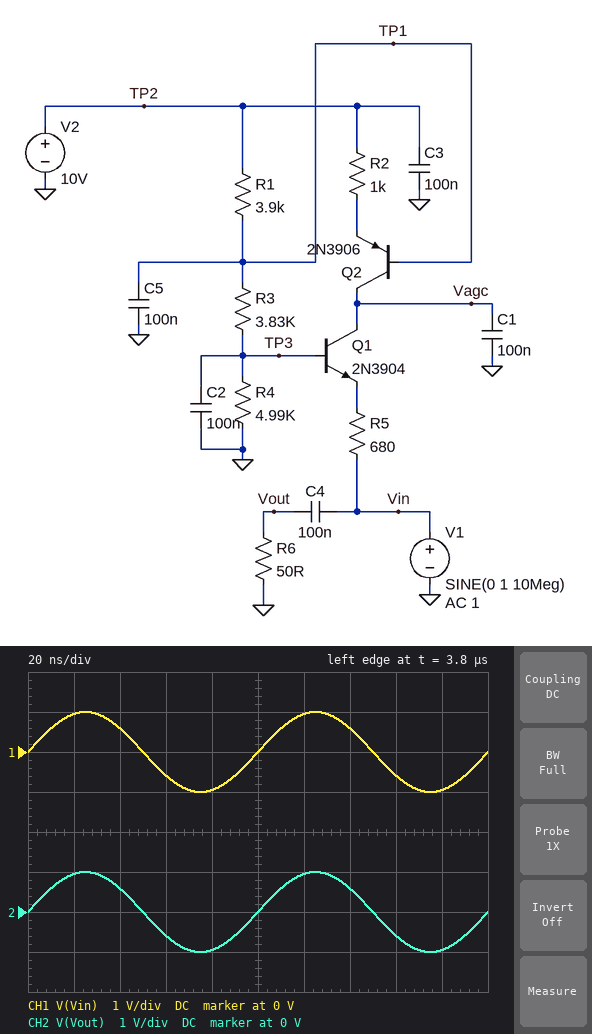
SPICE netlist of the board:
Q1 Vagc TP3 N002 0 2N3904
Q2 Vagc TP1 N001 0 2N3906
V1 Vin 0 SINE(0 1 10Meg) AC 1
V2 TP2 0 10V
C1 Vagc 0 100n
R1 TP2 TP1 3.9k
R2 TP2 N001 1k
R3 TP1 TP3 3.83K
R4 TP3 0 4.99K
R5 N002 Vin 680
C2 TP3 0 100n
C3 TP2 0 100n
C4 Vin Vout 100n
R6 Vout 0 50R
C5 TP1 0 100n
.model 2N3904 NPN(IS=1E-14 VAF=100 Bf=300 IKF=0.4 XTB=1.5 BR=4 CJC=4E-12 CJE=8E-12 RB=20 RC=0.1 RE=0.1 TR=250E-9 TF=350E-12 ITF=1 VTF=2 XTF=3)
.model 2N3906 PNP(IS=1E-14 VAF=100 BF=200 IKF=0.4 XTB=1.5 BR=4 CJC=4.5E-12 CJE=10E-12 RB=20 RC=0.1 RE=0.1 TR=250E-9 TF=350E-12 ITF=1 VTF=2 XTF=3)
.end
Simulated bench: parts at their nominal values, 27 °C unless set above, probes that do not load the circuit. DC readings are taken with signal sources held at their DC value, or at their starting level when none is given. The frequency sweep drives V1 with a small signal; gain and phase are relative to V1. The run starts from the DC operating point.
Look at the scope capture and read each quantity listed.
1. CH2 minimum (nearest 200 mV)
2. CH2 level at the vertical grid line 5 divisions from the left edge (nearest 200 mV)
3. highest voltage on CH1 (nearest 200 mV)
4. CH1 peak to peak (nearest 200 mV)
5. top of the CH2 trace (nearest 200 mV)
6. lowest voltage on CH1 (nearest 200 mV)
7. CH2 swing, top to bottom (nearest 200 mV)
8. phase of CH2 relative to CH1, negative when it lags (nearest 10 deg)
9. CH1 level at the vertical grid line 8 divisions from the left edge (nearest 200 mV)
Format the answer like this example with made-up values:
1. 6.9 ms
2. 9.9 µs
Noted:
1. -1.0 V
2. 0 V
3. 1.0 V
4. 2.0 V
5. 1.0 V
6. -1.0 V
7. 2.0 V
8. 0 deg
9. -600 mV
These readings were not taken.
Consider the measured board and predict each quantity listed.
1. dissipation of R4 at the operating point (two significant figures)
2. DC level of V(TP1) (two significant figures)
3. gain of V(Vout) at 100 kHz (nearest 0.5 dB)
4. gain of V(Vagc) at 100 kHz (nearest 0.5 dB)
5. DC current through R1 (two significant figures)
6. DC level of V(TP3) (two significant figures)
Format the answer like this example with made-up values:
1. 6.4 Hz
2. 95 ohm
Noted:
1. 1.7 mW
2. 6.4 V
3. -0.5 dB
4. -33.5 dB
5. 910 µA
6. 2.9 V
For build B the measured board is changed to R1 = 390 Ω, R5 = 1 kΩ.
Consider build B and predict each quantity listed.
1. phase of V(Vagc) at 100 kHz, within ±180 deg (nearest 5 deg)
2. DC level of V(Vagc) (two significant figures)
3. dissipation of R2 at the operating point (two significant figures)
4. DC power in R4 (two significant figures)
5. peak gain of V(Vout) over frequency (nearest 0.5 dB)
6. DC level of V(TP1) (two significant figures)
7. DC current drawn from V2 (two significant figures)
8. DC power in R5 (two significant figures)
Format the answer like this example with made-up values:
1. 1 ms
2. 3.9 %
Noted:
1. -75 deg
2. 1.5 V
3. 14 µW
4. 1.0 mW
5. 0 dB
6. 9.3 V
7. 2.0 mA
8. 2.3 mW
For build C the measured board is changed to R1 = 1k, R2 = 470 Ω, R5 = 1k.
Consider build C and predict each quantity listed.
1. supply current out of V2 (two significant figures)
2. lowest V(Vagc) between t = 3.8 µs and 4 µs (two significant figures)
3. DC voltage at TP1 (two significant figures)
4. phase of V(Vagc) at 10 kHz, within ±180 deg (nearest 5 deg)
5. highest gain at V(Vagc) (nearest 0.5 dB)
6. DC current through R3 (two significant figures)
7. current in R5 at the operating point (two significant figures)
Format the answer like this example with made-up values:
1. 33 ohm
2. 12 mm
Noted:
1. 3.0 mA
2. 2.4 V
3. 8.6 V
4. -75 deg
5. -5.0 dB
6. 1.4 mA
7. 2.4 mA
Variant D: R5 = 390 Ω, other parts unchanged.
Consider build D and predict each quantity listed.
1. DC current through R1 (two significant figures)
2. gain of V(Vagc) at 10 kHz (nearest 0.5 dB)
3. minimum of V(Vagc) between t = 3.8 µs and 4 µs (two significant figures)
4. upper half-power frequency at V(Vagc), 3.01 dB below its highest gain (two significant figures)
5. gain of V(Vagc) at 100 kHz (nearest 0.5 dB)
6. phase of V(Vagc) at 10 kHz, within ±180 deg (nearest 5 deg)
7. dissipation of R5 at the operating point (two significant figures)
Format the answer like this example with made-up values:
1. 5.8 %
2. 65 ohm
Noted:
1. 1.0 mA
2. -13.5 dB
3. 1.5 V
4. 2.9 kHz
5. -29.0 dB
6. -65 deg
7. 5.6 mW
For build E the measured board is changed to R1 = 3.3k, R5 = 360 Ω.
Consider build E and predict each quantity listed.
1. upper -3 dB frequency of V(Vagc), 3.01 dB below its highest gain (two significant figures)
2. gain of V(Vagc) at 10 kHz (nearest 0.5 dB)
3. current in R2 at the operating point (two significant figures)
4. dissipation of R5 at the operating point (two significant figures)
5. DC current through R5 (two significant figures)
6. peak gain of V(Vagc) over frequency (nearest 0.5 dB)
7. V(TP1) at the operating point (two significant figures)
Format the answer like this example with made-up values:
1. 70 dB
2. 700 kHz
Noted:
1. 3.1 kHz
2. -13.0 dB
3. 3.0 mA
4. 4.9 mW
5. 3.7 mA
6. -2.0 dB
7. 6.3 V
